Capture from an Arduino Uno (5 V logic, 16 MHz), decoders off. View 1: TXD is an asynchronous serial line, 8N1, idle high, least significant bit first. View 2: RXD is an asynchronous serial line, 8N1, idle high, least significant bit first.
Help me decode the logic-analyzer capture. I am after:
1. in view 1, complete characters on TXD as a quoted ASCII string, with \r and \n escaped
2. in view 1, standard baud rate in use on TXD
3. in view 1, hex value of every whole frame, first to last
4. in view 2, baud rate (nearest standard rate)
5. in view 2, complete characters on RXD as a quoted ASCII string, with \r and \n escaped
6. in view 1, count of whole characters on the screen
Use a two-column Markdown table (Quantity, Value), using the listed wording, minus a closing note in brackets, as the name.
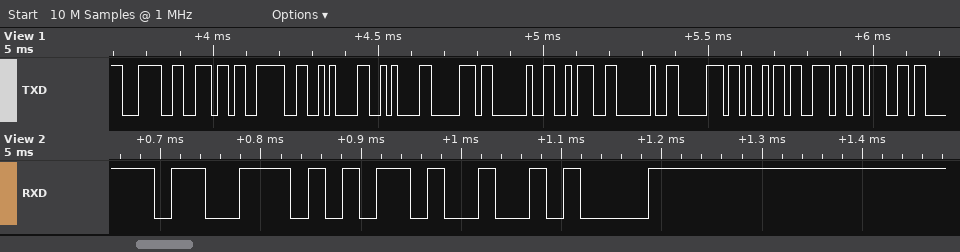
| Quantity | Value |
|---|---|
| in view 1, complete characters on TXD as a quoted ASCII string, with \r and \n escaped | "<n>\n\np : ping" |
| in view 1, standard baud rate in use on TXD | 57600 baud |
| in view 1, hex value of every whole frame, first to last | 3C 6E 3E 0A 0A 70 20 3A 20 70 69 6E 67 |
| in view 2, baud rate | 57600 baud |
| in view 2, complete characters on RXD as a quoted ASCII string, with \r and \n escaped | "s-\n" |
| in view 1, count of whole characters on the screen | 13 |
